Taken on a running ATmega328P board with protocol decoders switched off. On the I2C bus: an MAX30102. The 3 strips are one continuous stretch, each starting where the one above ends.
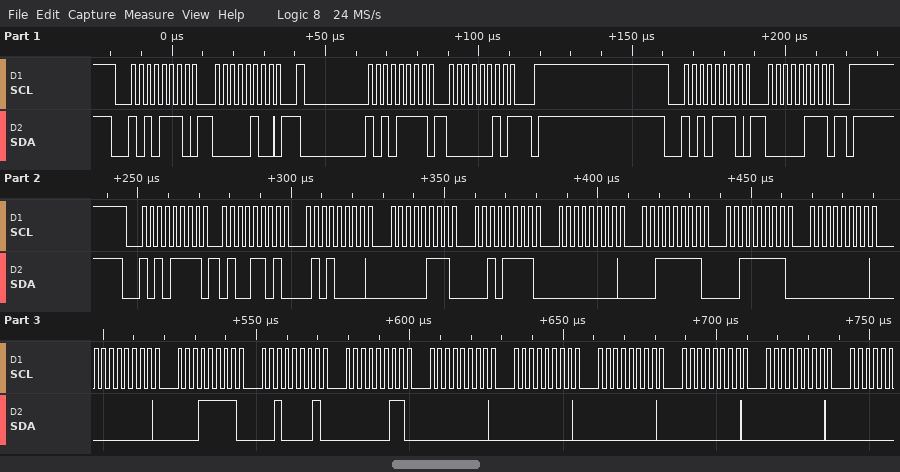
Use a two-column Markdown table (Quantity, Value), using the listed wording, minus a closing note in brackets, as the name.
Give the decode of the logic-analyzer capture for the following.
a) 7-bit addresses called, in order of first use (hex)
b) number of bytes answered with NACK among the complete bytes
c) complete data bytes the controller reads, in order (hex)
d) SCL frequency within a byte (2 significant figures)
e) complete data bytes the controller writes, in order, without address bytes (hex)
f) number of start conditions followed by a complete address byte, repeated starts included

| Quantity | Value |
|---|---|
| 7-bit addresses called, in order of first use | 0x57 |
| number of bytes answered with NACK among the complete bytes | 1 |
| complete data bytes the controller reads, in order | 02 4D 50 07 2F 00 3F 3F 00 00 1F 21 03 00 00 00 00 00 |
| SCL frequency within a byte | 400 kHz |
| complete data bytes the controller writes, in order, without address bytes | 04 07 |
| number of start conditions followed by a complete address byte, repeated starts included | 4 |
